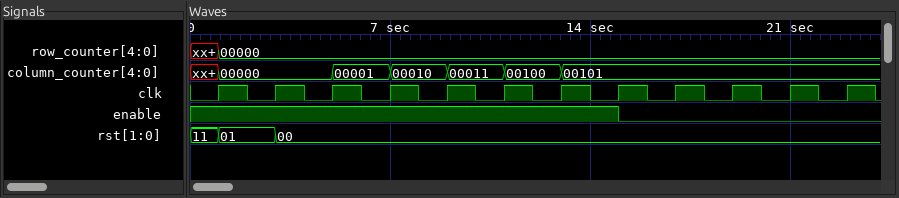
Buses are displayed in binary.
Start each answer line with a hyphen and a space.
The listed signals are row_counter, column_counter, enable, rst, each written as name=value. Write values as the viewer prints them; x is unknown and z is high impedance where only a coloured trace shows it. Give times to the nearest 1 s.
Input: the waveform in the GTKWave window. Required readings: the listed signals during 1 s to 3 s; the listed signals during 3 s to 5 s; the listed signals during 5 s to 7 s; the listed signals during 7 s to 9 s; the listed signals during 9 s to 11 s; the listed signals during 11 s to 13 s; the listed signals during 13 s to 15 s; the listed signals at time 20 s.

- row_counter=00000, column_counter=00000, enable=1, rst=01
- row_counter=00000, column_counter=00000, enable=1, rst=00
- row_counter=00000, column_counter=00001, enable=1, rst=00
- row_counter=00000, column_counter=00010, enable=1, rst=00
- row_counter=00000, column_counter=00011, enable=1, rst=00
- row_counter=00000, column_counter=00100, enable=1, rst=00
- row_counter=00000, column_counter=00101, enable=1, rst=00
- row_counter=00000, column_counter=00101, enable=0, rst=00
